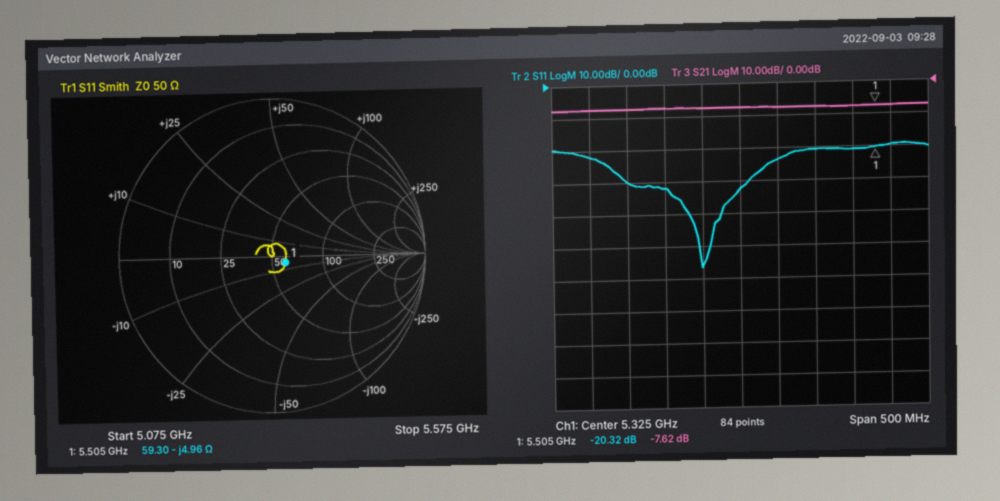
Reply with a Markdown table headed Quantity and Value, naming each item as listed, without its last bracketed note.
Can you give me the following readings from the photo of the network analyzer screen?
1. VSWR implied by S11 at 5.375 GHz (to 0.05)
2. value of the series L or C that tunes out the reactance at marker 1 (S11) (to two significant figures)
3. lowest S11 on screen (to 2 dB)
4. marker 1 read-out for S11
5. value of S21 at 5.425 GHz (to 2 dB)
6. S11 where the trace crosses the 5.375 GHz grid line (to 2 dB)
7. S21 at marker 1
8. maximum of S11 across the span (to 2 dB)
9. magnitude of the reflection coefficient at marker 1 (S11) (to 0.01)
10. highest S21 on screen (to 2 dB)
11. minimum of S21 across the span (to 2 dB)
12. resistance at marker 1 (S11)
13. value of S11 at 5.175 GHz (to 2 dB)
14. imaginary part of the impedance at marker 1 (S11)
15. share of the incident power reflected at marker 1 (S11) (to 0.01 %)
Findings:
| Quantity | Value |
|---|---|
| VSWR implied by S11 at 5.375 GHz | 1.15 |
| value of the series L or C that tunes out the reactance at marker 1 (S11) | 140 pH |
| lowest S11 on screen | -56 dB |
| marker 1 read-out for S11 | -20.32 dB |
| value of S21 at 5.425 GHz | -8 dB |
| S11 where the trace crosses the 5.375 GHz grid line | -24 dB |
| S21 at marker 1 | -7.62 dB |
| maximum of S11 across the span | -20 dB |
| magnitude of the reflection coefficient at marker 1 (S11) | 0.10 |
| highest S21 on screen | -8 dB |
| minimum of S21 across the span | -8 dB |
| resistance at marker 1 | 59.30 Ω |
| value of S11 at 5.175 GHz | -30 dB |
| imaginary part of the impedance at marker 1 | -4.96 Ω |
| share of the incident power reflected at marker 1 (S11) | 0.93 % |
